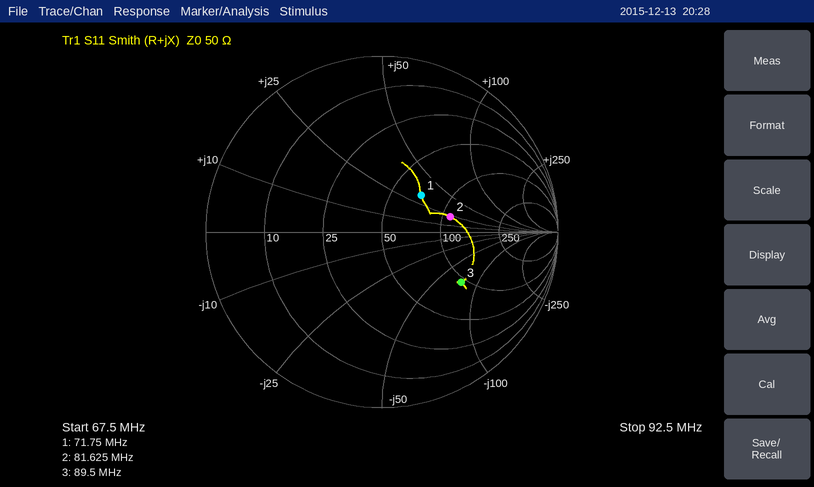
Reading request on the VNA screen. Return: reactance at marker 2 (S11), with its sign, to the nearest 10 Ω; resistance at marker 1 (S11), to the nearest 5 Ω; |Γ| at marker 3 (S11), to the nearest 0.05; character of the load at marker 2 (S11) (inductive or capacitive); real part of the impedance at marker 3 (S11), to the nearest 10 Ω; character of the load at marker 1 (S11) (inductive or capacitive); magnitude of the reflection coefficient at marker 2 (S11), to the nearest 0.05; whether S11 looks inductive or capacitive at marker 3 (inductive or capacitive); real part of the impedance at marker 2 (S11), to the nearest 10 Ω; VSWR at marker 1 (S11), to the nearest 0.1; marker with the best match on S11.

+20 Ω
70 Ω
0.55
inductive
90 Ω
inductive
0.40
capacitive
110 Ω
1.9
marker 1
